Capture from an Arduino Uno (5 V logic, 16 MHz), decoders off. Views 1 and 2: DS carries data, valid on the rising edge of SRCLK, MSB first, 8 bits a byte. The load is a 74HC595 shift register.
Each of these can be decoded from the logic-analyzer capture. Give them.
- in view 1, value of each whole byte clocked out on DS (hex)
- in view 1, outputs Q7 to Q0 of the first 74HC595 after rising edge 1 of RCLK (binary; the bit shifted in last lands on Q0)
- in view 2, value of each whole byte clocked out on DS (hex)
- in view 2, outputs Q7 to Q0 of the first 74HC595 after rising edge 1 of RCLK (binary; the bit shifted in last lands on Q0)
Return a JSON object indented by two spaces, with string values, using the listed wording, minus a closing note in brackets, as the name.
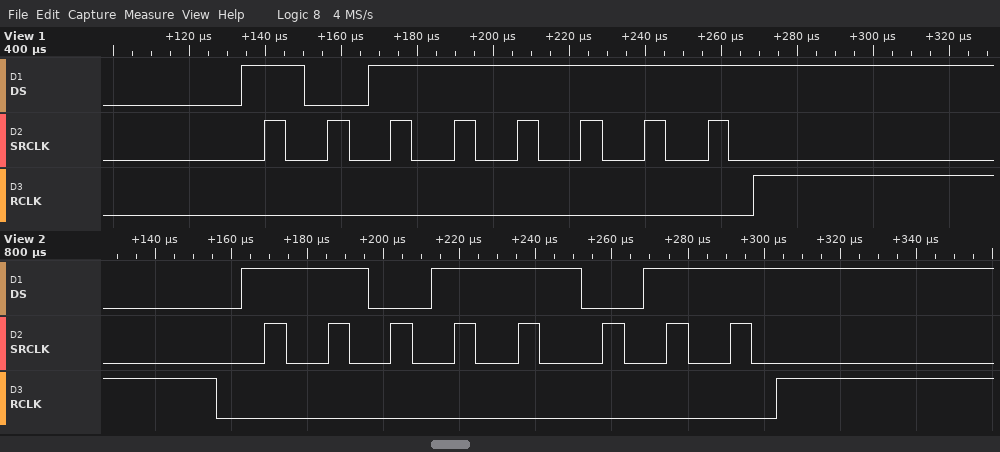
{
  "in view 1, value of each whole byte clocked out on DS": "0xBF",
  "in view 1, outputs Q7 to Q0 of the first 74HC595 after rising edge 1 of RCLK": "10111111",
  "in view 2, value of each whole byte clocked out on DS": "DB",
  "in view 2, outputs Q7 to Q0 of the first 74HC595 after rising edge 1 of RCLK": "11011011"
}
